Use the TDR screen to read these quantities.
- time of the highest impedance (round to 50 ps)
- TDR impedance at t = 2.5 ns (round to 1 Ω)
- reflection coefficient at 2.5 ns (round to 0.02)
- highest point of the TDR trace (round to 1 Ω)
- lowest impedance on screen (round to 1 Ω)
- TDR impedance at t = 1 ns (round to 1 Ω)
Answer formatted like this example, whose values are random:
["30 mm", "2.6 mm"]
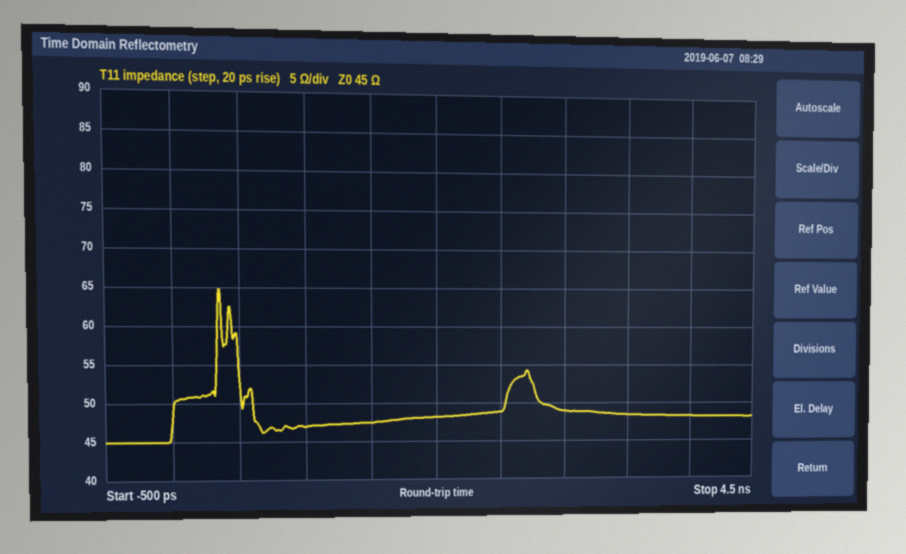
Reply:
["350 ps", "49 Ω", "+0.04", "65 Ω", "45 Ω", "47 Ω"]
